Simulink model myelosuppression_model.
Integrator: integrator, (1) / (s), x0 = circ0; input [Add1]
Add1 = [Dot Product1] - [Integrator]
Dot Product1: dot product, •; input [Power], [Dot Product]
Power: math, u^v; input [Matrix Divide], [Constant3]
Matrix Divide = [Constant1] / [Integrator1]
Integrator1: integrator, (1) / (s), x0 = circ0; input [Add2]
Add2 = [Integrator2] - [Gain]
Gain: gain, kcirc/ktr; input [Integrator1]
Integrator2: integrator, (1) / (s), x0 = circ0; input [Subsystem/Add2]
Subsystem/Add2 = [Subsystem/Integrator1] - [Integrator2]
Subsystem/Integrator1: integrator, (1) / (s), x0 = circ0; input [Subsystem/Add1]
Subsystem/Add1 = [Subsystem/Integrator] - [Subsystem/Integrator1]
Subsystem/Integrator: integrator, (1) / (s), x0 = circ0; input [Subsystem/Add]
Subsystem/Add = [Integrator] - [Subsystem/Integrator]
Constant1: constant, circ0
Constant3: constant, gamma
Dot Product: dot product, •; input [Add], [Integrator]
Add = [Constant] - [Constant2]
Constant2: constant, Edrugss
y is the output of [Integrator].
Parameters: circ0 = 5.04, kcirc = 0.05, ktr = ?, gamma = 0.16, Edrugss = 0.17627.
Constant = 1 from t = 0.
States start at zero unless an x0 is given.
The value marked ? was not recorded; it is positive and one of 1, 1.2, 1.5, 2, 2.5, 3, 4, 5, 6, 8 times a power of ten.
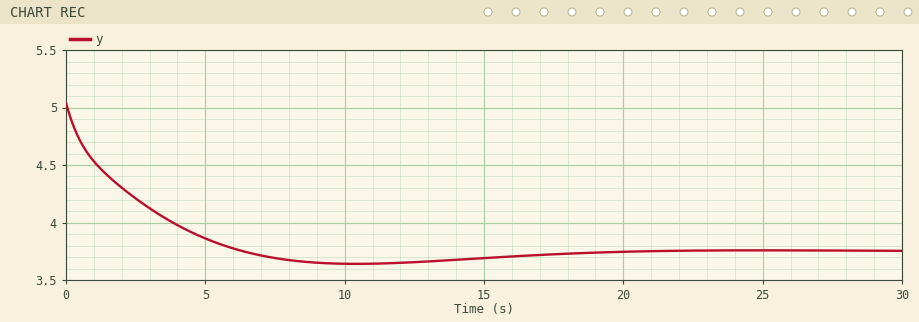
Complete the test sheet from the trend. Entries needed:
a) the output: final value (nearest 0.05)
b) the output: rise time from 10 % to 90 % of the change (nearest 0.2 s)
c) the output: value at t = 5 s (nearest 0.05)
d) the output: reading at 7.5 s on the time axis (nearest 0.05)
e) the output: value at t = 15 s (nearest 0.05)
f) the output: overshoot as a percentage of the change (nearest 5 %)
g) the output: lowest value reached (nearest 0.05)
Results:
3.75
4.6 s
3.85
3.70
3.70
10 %
3.65
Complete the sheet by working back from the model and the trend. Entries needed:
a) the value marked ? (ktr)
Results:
0.02
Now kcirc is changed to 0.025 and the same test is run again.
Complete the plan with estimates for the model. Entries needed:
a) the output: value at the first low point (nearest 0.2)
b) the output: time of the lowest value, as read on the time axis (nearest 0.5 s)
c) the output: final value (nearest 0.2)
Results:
1.6
12.5 s
1.8
